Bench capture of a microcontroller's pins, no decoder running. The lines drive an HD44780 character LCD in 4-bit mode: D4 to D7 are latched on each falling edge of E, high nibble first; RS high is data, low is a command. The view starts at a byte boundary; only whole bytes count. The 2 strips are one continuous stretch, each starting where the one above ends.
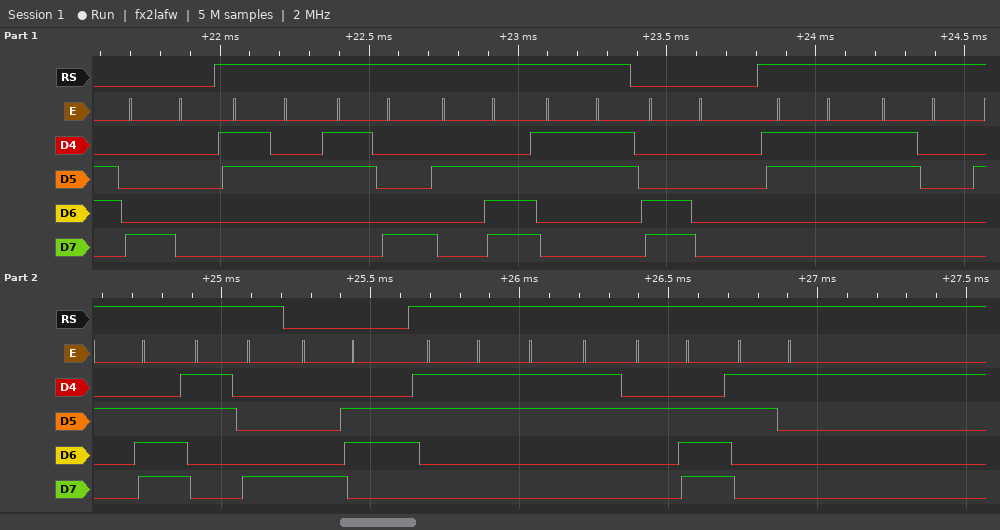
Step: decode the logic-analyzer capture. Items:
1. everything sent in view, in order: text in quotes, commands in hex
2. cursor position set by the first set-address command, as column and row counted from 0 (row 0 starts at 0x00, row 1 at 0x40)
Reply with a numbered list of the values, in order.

1. 0x80 "28.3" 0xC0 "30.8" 0x86 "33.1"
2. column 0, row 0
